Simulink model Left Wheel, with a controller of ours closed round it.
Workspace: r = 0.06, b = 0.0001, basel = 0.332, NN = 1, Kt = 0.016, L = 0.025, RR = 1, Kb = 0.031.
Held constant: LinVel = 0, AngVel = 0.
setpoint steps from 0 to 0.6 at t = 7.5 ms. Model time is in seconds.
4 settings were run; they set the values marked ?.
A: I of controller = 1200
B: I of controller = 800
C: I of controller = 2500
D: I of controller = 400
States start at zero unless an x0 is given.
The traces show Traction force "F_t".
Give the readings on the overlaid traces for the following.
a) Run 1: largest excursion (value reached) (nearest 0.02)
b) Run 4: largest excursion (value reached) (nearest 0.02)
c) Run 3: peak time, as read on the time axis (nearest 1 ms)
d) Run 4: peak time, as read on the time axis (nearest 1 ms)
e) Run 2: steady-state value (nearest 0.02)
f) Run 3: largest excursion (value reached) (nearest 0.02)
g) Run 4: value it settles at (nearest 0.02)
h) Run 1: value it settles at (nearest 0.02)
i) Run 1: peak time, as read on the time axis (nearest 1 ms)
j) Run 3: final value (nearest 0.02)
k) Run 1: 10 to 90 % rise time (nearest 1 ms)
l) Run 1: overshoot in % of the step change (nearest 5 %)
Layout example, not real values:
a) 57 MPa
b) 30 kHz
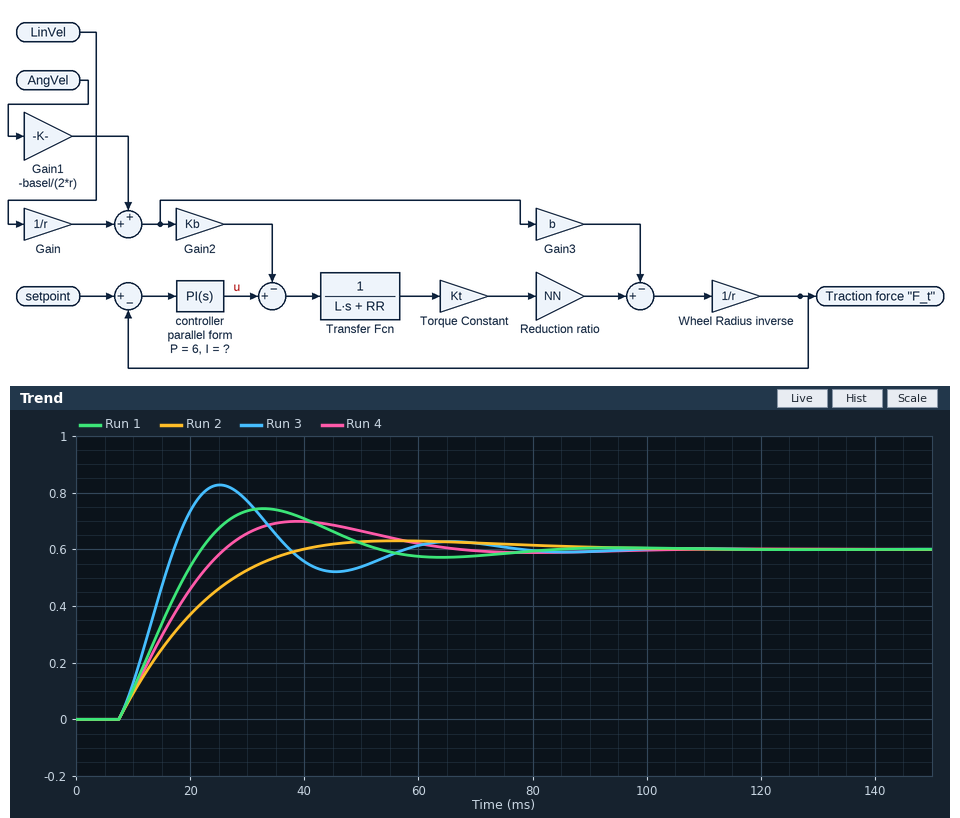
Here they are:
a) 0.74
b) 0.70
c) 25 ms
d) 39 ms
e) 0.60
f) 0.82
g) 0.60
h) 0.60
i) 33 ms
j) 0.60
k) 11 ms
l) 25 %
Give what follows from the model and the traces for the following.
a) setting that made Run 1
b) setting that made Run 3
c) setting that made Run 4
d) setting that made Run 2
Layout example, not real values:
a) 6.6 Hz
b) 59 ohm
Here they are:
a) A
b) C
c) B
d) D
